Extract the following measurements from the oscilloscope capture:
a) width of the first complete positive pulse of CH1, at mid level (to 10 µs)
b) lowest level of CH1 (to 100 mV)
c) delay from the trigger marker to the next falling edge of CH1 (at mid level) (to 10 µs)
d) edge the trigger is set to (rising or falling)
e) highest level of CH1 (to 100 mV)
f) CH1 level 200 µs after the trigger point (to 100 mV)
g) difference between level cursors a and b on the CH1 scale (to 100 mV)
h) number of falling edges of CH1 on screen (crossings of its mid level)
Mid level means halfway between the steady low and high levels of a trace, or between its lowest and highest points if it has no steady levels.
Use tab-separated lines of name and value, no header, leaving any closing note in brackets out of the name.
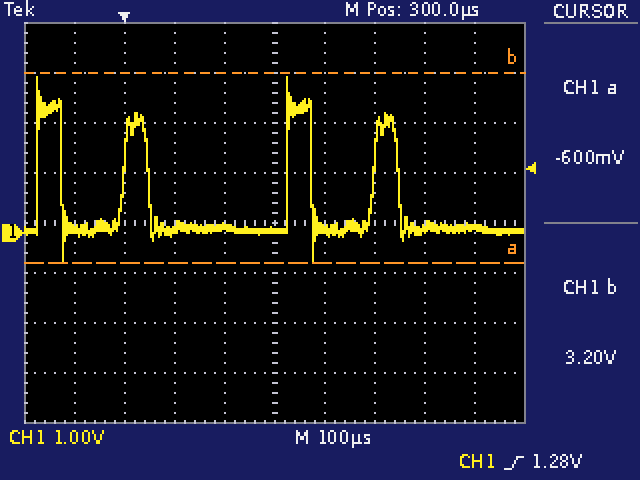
width of the first complete positive pulse of CH1, at mid level	50 µs
lowest level of CH1	-600 mV
delay from the trigger marker to the next falling edge of CH1 (at mid level)	50 µs
edge the trigger is set to	rising
highest level of CH1	3.1 V
CH1 level 200 µs after the trigger point	100 mV
difference between level cursors a and b on the CH1 scale	3.8 V
number of falling edges of CH1 on screen	4
